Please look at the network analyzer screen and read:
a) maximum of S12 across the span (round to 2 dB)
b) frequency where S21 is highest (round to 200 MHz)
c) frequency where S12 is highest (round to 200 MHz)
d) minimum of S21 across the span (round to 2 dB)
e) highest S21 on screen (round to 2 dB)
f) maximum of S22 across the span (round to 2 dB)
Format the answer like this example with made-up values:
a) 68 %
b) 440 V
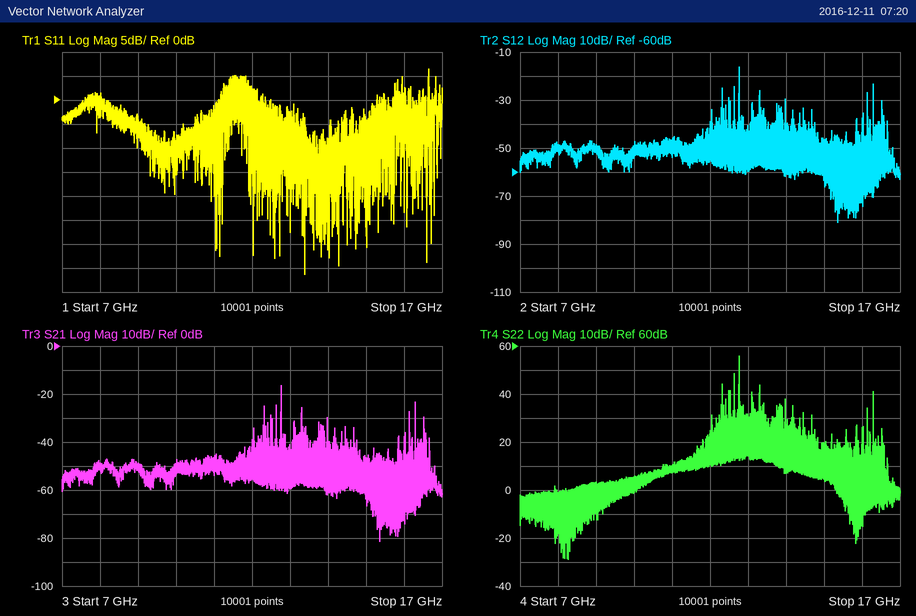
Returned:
a) -16 dB
b) 12.8 GHz
c) 12.8 GHz
d) -82 dB
e) -16 dB
f) 56 dB
